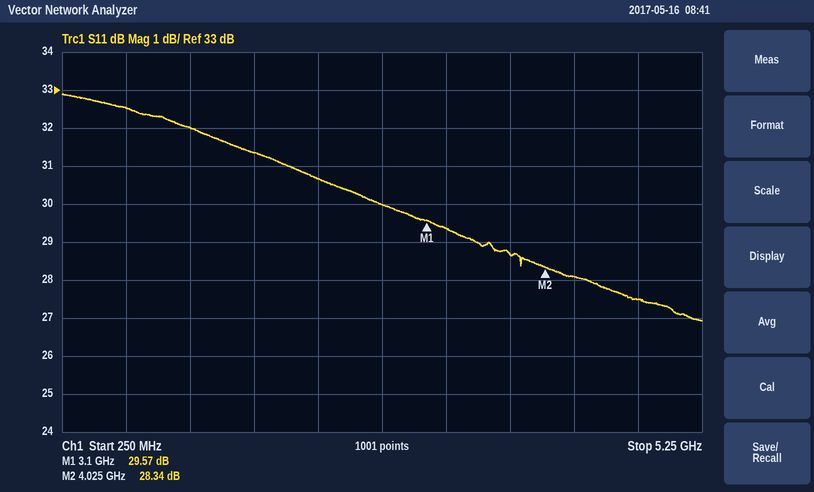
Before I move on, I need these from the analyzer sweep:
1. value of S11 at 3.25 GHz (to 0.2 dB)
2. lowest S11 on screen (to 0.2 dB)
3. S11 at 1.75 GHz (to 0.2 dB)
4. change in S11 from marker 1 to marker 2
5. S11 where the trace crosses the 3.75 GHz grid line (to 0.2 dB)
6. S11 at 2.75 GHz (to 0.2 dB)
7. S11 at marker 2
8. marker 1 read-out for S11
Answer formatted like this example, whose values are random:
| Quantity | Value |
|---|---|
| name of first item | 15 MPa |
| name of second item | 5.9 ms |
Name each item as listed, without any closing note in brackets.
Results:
| Quantity | Value |
|---|---|
| value of S11 at 3.25 GHz | 29.4 dB |
| lowest S11 on screen | 27.0 dB |
| S11 at 1.75 GHz | 31.4 dB |
| change in S11 from marker 1 to marker 2 | -1.23 dB |
| S11 where the trace crosses the 3.75 GHz grid line | 28.6 dB |
| S11 at 2.75 GHz | 30.0 dB |
| S11 at marker 2 | 28.34 dB |
| marker 1 read-out for S11 | 29.57 dB |
